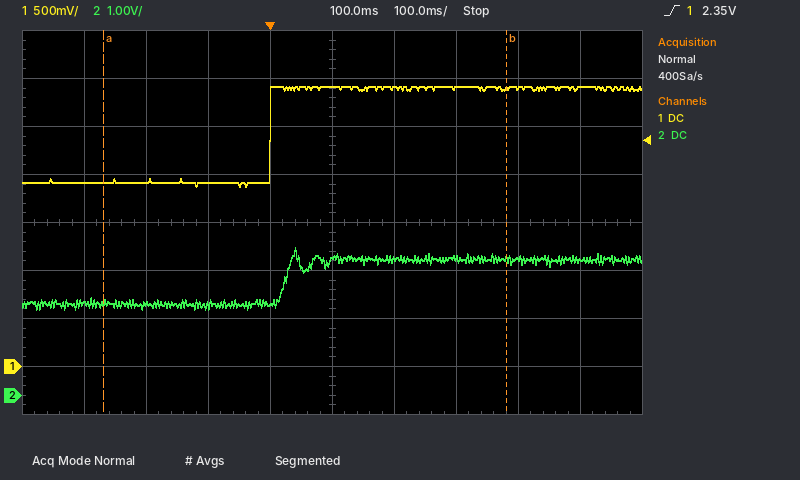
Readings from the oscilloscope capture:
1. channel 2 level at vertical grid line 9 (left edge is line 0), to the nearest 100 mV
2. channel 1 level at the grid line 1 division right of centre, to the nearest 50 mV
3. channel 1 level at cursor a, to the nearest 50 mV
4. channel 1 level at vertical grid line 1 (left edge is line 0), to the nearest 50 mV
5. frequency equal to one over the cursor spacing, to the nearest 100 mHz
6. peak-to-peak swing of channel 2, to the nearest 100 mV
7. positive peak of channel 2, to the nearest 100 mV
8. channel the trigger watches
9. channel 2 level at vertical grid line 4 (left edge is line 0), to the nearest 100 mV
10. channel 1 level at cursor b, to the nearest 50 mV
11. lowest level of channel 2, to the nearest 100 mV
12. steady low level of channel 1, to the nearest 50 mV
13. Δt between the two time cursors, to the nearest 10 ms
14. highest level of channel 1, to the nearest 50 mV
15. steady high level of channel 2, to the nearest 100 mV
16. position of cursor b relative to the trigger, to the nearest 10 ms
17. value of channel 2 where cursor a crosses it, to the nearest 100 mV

2.8 V
2.90 V
1.90 V
1.90 V
1.5 Hz
1.3 V
3.1 V
channel 1
1.9 V
2.90 V
1.8 V
1.90 V
650 ms
2.90 V
2.8 V
+380 ms
1.9 V
